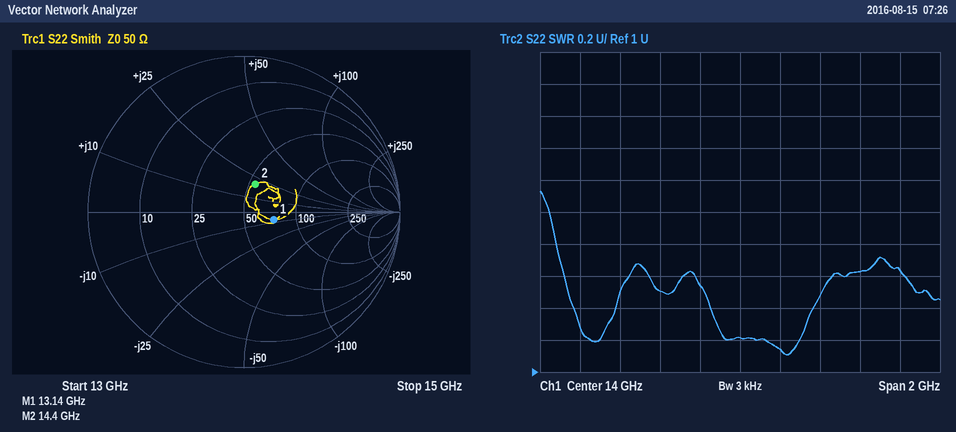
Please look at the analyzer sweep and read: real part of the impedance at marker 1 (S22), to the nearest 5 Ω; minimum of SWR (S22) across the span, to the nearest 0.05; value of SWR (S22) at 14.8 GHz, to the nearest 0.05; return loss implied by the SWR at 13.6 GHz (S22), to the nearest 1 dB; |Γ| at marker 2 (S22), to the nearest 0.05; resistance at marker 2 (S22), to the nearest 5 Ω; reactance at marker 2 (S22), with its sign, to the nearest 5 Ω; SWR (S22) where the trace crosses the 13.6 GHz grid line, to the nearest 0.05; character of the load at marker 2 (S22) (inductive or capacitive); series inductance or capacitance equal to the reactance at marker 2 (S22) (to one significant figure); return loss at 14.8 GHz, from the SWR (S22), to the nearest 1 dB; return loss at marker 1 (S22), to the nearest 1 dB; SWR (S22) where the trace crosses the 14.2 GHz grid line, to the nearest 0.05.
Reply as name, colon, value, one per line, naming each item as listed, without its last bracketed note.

real part of the impedance at marker 1 (S22), to the nearest 5 Ω: 75 Ω
minimum of SWR (S22) across the span, to the nearest 0.05: 1.10
value of SWR (S22) at 14.8 GHz, to the nearest 0.05: 1.65
return loss implied by the SWR at 13.6 GHz (S22), to the nearest 1 dB: 14 dB
|Γ| at marker 2 (S22), to the nearest 0.05: 0.20
resistance at marker 2 (S22), to the nearest 5 Ω: 55 Ω
reactance at marker 2 (S22), with its sign, to the nearest 5 Ω: +20 Ω
SWR (S22) where the trace crosses the 13.6 GHz grid line, to the nearest 0.05: 1.50
character of the load at marker 2 (S22): inductive
series inductance or capacitance equal to the reactance at marker 2 (S22): 200 pH
return loss at 14.8 GHz, from the SWR (S22), to the nearest 1 dB: 12 dB
return loss at marker 1 (S22), to the nearest 1 dB: 14 dB
SWR (S22) where the trace crosses the 14.2 GHz grid line, to the nearest 0.05: 1.15
